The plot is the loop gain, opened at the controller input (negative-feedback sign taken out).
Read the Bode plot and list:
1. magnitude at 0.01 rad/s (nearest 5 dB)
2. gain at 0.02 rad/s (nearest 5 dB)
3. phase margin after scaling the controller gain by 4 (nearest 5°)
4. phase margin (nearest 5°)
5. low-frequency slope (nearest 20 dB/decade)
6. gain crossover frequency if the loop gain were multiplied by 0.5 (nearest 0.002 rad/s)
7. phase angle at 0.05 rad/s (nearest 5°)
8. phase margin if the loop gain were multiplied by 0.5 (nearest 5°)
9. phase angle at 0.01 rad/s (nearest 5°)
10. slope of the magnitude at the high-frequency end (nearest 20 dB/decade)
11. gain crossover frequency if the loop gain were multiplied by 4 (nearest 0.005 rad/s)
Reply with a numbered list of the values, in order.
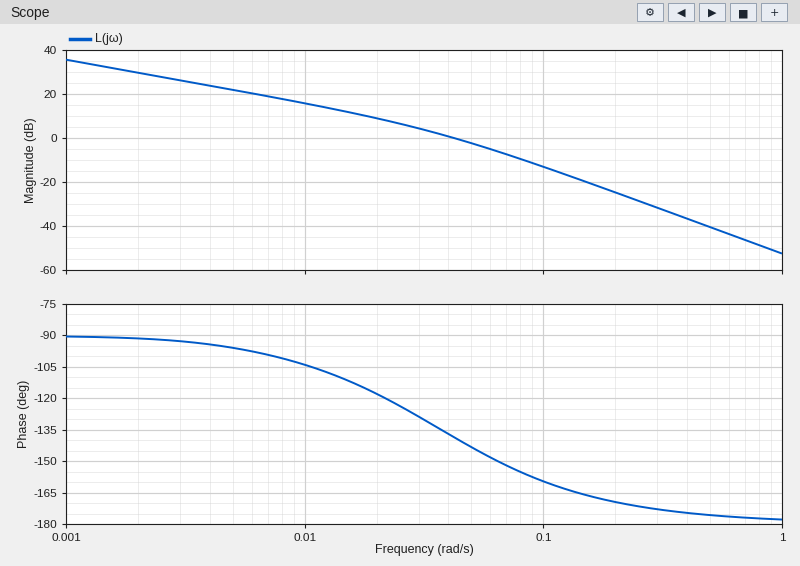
1. 15 dB
2. 10 dB
3. 20°
4. 40°
5. -20 dB/decade
6. 0.026 rad/s
7. -145°
8. 55°
9. -105°
10. -40 dB/decade
11. 0.095 rad/s
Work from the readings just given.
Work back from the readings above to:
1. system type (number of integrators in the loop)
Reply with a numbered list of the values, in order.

1. 1
